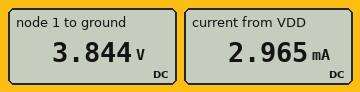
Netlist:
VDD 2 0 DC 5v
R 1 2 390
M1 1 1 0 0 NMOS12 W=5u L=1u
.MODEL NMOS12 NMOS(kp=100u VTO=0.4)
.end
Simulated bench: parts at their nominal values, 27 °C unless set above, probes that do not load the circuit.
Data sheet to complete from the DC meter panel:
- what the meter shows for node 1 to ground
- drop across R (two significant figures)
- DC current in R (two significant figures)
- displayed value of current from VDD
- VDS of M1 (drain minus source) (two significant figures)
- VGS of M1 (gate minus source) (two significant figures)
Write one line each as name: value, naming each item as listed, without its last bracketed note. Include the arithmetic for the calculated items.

what the meter shows for node 1 to ground: 3.844 V
drop across R: 5 V - 3.844 V = 1.2 V
DC current in R: (5 V - 3.844 V) / 390 Ω = 3.0 mA
displayed value of current from VDD: 2.965 mA
VDS of M1 (drain minus source): 3.844 V = 3.8 V
VGS of M1 (gate minus source): 3.844 V = 3.8 V
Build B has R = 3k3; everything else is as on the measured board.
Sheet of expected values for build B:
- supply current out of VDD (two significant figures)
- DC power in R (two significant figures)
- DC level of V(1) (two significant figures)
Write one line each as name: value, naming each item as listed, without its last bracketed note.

supply current out of VDD: 840 µA
DC power in R: 2.3 mW
DC level of V(1): 2.2 V
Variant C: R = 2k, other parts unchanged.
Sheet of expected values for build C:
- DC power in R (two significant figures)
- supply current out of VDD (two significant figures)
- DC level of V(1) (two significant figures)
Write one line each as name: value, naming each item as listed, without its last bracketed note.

DC power in R: 2.9 mW
supply current out of VDD: 1.2 mA
DC level of V(1): 2.6 V
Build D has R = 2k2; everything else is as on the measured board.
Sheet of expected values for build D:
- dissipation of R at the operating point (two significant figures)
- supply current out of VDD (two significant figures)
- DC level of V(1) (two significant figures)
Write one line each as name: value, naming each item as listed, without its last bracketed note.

dissipation of R at the operating point: 2.8 mW
supply current out of VDD: 1.1 mA
DC level of V(1): 2.5 V
